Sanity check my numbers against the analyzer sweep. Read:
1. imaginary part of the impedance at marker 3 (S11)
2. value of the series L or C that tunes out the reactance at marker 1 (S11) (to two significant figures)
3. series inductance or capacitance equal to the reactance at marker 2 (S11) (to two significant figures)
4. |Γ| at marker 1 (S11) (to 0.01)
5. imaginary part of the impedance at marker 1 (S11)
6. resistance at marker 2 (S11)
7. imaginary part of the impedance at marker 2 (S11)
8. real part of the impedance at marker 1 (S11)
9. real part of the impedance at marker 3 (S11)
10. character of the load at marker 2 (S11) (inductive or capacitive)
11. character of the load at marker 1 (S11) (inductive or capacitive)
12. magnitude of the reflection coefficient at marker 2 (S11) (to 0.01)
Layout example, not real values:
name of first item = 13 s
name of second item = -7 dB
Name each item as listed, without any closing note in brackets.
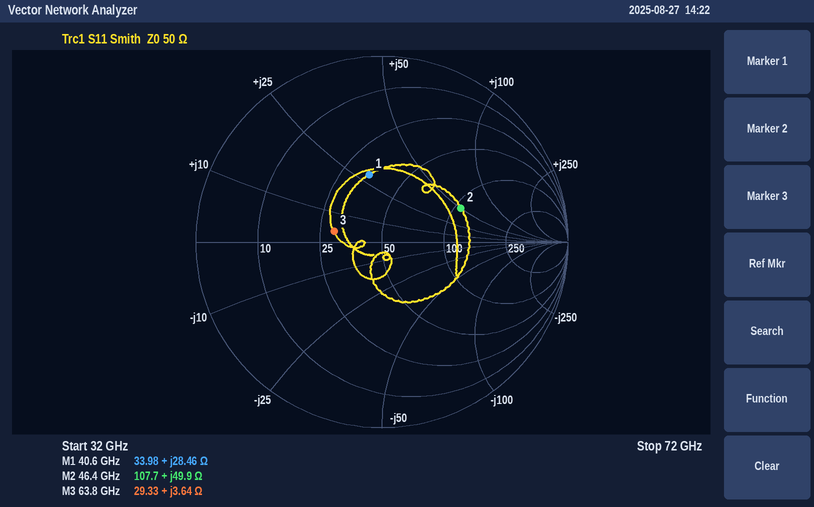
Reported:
imaginary part of the impedance at marker 3 = +3.64 Ω
value of the series L or C that tunes out the reactance at marker 1 (S11) = 140 fF
series inductance or capacitance equal to the reactance at marker 2 (S11) = 170 pH
|Γ| at marker 1 (S11) = 0.37
imaginary part of the impedance at marker 1 = +28.46 Ω
resistance at marker 2 = 107.7 Ω
imaginary part of the impedance at marker 2 = +49.9 Ω
real part of the impedance at marker 1 = 33.98 Ω
real part of the impedance at marker 3 = 29.33 Ω
character of the load at marker 2 (S11) = inductive
character of the load at marker 1 (S11) = inductive
magnitude of the reflection coefficient at marker 2 (S11) = 0.46
